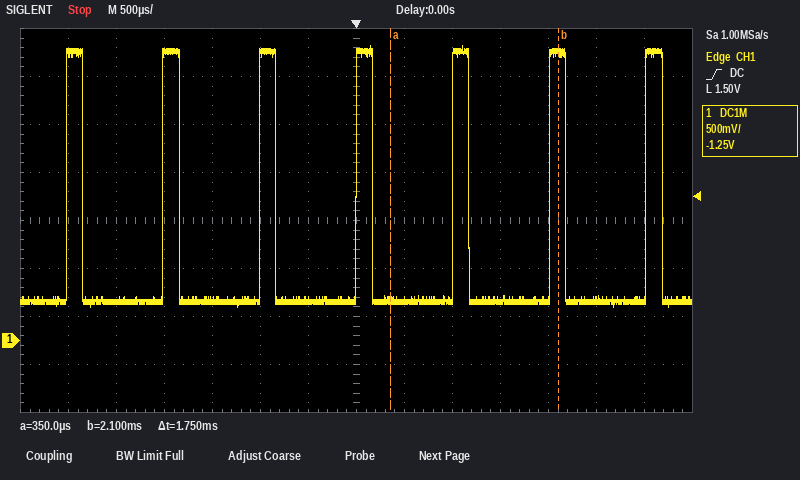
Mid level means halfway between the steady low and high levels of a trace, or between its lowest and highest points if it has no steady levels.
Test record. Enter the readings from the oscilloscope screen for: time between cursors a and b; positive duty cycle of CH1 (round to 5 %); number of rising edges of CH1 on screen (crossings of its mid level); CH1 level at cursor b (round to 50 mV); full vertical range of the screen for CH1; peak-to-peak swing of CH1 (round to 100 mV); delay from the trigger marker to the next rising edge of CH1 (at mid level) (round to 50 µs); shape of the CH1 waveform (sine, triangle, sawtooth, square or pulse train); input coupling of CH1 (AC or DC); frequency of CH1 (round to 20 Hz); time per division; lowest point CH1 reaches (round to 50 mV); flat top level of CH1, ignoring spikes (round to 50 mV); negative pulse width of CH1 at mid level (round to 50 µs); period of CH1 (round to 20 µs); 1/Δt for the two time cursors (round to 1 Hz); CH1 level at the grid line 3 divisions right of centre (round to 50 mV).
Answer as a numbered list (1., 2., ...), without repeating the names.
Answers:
1. 1.75 ms
2. 15 %
3. 7
4. 3.00 V
5. 4 V
6. 2.70 V
7. 1.00 ms
8. pulse train
9. DC
10. 1.00 kHz
11. 500 µs
12. 350 mV
13. 3.00 V
14. 850 µs
15. 1.00 ms
16. 571 Hz
17. 400 mV
